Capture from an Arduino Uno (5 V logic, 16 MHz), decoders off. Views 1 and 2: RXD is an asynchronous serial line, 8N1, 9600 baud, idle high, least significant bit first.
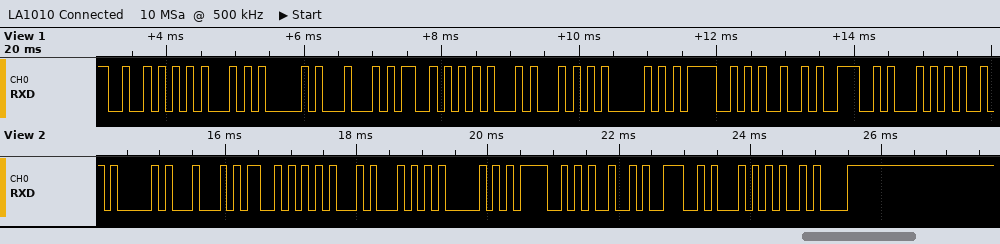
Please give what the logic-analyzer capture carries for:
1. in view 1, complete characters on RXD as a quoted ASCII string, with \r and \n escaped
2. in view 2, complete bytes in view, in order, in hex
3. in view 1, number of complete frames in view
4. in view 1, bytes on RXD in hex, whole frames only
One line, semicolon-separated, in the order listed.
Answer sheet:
"READSETPOINT"; 41 44 53 45 54 50 4F 49 4E 54 0A; 12; 0x52 0x45 0x41 0x44 0x53 0x45 0x54 0x50 0x4F 0x49 0x4E 0x54
